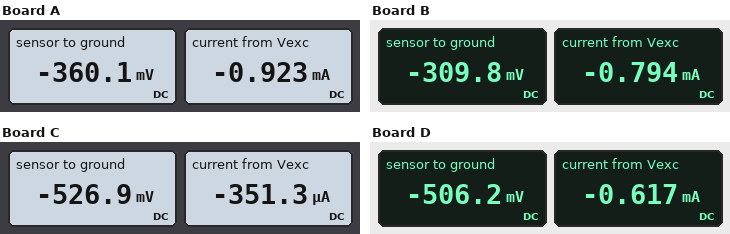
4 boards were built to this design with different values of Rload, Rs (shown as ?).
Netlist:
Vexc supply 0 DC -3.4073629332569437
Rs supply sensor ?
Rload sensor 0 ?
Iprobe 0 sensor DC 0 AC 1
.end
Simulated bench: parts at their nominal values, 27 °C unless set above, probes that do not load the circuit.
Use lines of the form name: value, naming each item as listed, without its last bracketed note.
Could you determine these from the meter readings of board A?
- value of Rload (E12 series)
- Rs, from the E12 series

value of Rload: 390 Ω
Rs, from the E12 series: 3.3 kΩ
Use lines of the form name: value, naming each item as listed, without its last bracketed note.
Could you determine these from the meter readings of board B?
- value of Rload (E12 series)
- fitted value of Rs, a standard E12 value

value of Rload: 390 Ω
fitted value of Rs, a standard E12 value: 3.9 kΩ
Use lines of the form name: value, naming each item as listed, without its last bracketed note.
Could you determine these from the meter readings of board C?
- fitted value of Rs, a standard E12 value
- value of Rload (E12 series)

fitted value of Rs, a standard E12 value: 8.2 kΩ
value of Rload: 1.5 kΩ
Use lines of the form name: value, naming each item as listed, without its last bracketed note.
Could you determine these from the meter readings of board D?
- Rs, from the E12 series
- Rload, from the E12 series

Rs, from the E12 series: 4.7 kΩ
Rload, from the E12 series: 820 Ω
